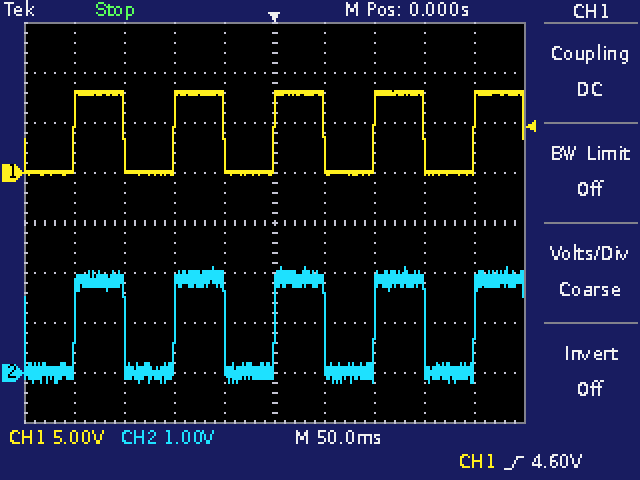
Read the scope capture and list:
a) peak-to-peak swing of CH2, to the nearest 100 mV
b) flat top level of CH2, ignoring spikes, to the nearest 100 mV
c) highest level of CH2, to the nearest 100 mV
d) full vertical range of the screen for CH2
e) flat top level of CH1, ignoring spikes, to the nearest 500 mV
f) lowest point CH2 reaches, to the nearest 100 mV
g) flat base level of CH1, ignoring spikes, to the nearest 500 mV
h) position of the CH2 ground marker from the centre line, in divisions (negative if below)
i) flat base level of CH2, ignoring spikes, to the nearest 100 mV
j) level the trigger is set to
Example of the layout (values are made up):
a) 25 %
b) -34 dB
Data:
a) 2.3 V
b) 1.9 V
c) 2.1 V
d) 8 V
e) 8.0 V
f) -200 mV
g) 0.0 V
h) -3.0 div
i) 0.0 V
j) 4.60 V
